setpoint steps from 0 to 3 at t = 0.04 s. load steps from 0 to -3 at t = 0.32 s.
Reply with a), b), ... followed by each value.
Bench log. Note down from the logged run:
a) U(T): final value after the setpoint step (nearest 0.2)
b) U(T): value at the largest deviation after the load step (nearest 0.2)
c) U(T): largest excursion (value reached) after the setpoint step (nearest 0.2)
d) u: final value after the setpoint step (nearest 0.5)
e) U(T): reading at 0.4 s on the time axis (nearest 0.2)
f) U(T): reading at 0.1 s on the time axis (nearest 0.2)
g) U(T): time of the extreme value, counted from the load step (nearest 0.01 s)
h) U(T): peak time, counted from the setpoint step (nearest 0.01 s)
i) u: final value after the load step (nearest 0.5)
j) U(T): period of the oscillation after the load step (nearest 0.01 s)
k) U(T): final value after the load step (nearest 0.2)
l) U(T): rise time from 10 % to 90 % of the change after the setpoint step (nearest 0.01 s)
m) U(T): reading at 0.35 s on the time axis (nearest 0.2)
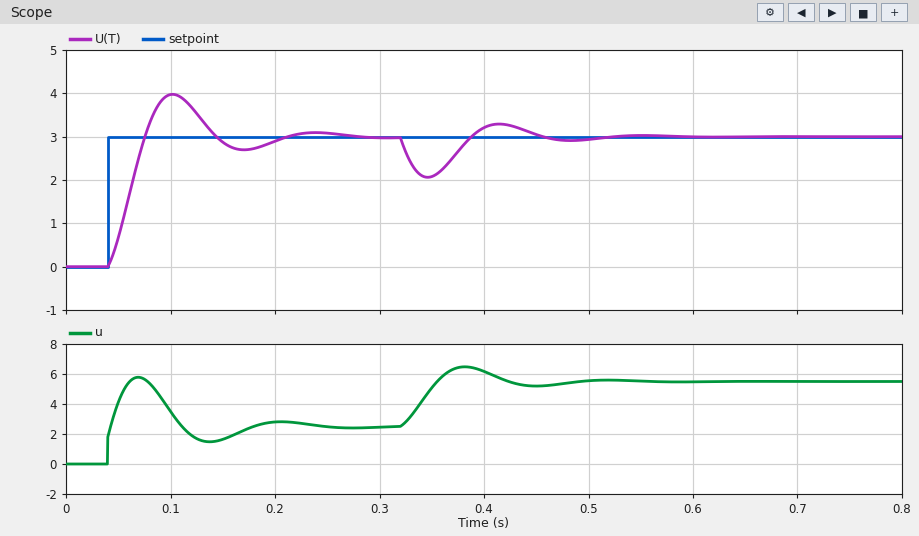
a) 3.0
b) 2.0
c) 4.0
d) 2.5
e) 3.2
f) 4.0
g) 0.03 s
h) 0.06 s
i) 5.5
j) 0.14 s
k) 3.0
l) 0.03 s
m) 2.0
